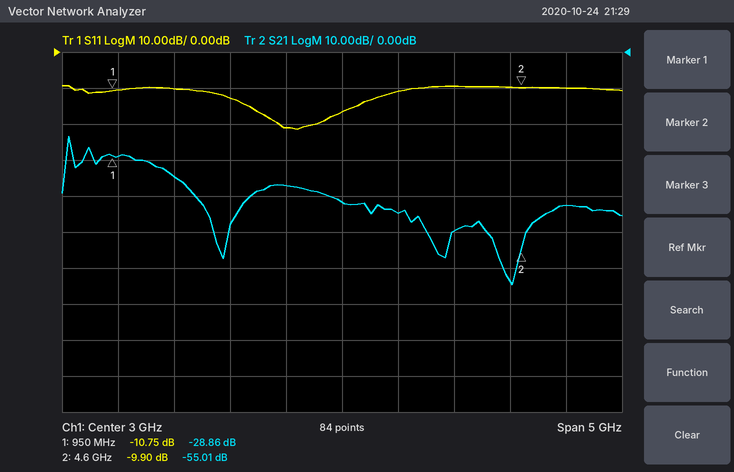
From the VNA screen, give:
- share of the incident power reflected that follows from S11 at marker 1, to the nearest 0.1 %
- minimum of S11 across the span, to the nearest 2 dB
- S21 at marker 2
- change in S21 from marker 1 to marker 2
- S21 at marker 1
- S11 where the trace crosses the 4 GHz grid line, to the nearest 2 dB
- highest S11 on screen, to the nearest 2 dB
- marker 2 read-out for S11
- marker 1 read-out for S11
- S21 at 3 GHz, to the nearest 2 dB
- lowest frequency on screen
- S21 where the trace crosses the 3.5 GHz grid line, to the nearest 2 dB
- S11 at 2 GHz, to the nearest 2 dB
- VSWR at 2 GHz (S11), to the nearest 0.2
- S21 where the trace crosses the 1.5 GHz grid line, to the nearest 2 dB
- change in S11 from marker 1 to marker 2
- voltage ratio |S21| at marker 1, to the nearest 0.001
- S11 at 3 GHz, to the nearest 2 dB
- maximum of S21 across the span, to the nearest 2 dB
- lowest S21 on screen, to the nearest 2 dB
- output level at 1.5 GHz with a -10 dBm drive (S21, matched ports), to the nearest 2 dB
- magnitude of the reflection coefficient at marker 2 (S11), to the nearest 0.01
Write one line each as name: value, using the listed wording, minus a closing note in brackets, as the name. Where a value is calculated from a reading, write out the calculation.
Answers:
share of the incident power reflected that follows from S11 at marker 1, to the nearest 0.1 %: 10^(-10.75/10) ≈ 8.4 %
minimum of S11 across the span, to the nearest 2 dB: -22 dB
S21 at marker 2: -55.01 dB
change in S21 from marker 1 to marker 2: -55.01 − (-28.86) = -26.15 dB
S21 at marker 1: -28.86 dB
S11 where the trace crosses the 4 GHz grid line, to the nearest 2 dB: -10 dB
highest S11 on screen, to the nearest 2 dB: -10 dB
marker 2 read-out for S11: -9.90 dB
marker 1 read-out for S11: -10.75 dB
S21 at 3 GHz, to the nearest 2 dB: -42 dB
lowest frequency on screen: 500 MHz
S21 where the trace crosses the 3.5 GHz grid line, to the nearest 2 dB: -44 dB
S11 at 2 GHz, to the nearest 2 dB: -12 dB
VSWR at 2 GHz (S11), to the nearest 0.2: |Γ| = 10^(-12/20) = 0.2512; VSWR = (1 + 0.2512)/(1 − 0.2512) ≈ 1.67, so 1.6 to the nearest 0.2
S21 where the trace crosses the 1.5 GHz grid line, to the nearest 2 dB: -34 dB
change in S11 from marker 1 to marker 2: -9.9 − (-10.75) = 0.85 dB
voltage ratio |S21| at marker 1, to the nearest 0.001: 10^(-28.86/20) ≈ 0.036
S11 at 3 GHz, to the nearest 2 dB: -16 dB
maximum of S21 across the span, to the nearest 2 dB: -24 dB
lowest S21 on screen, to the nearest 2 dB: -64 dB
output level at 1.5 GHz with a -10 dBm drive (S21, matched ports), to the nearest 2 dB: -10 dBm + (-34 dB) = -44 dBm
magnitude of the reflection coefficient at marker 2 (S11), to the nearest 0.01: 10^(-9.9/20) ≈ 0.32
